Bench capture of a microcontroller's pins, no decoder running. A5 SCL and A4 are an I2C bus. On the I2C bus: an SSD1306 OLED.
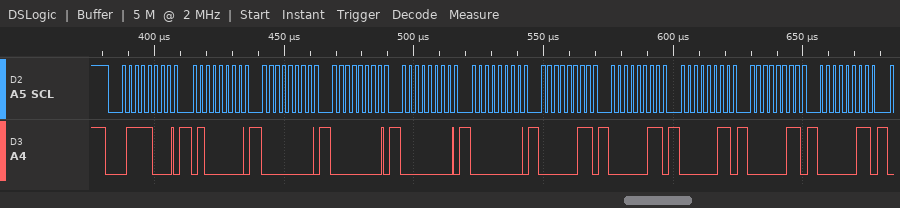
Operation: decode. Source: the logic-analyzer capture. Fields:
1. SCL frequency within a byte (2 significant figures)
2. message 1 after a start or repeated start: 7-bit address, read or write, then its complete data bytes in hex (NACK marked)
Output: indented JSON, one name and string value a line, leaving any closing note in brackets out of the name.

{
  "SCL frequency within a byte": "400 kHz",
  "message 1 after a start or repeated start: 7-bit address, read or write, then its complete data bytes in hex": "0x3C write: 40 00 00 00 00 03 03 03 03 03"
}
